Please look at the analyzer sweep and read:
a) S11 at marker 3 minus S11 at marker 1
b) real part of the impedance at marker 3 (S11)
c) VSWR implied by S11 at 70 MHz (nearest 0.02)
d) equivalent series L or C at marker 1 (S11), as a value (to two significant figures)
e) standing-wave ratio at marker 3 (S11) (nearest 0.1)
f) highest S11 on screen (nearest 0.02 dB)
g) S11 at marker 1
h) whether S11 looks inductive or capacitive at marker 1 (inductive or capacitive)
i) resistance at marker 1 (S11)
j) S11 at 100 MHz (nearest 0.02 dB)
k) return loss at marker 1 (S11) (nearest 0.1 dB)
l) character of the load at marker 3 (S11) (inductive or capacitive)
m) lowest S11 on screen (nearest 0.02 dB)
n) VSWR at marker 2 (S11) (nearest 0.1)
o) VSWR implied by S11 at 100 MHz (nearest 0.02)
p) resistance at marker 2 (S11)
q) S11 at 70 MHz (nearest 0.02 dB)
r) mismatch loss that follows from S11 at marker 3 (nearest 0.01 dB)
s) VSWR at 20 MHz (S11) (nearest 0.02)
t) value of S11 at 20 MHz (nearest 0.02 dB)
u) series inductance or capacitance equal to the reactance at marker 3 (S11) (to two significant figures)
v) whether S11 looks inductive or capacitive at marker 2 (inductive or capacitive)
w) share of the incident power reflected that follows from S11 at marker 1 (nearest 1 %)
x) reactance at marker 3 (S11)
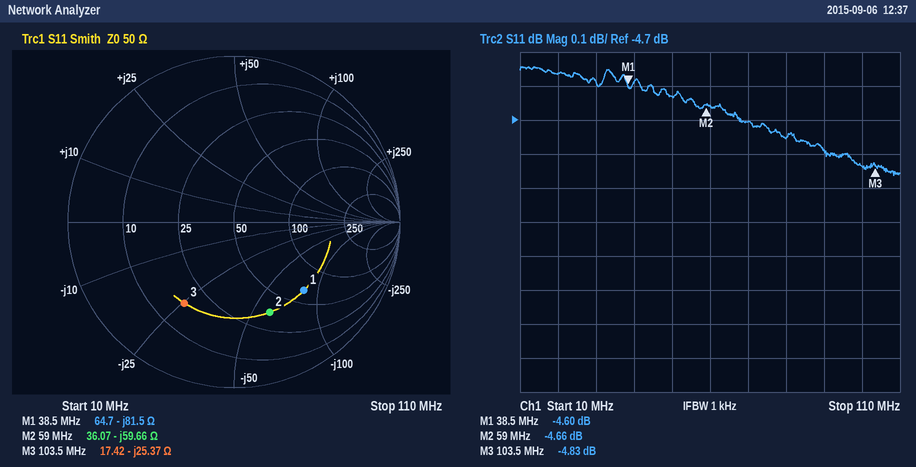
-0.23 dB
17.42 Ω
3.78
51 pF
3.7
-4.54 dB
-4.60 dB
capacitive
64.7 Ω
-4.84 dB
4.6 dB
capacitive
-4.86 dB
3.8
3.68
36.07 Ω
-4.70 dB
1.73 dB
3.90
-4.56 dB
61 pF
capacitive
35 %
-25.37 Ω
